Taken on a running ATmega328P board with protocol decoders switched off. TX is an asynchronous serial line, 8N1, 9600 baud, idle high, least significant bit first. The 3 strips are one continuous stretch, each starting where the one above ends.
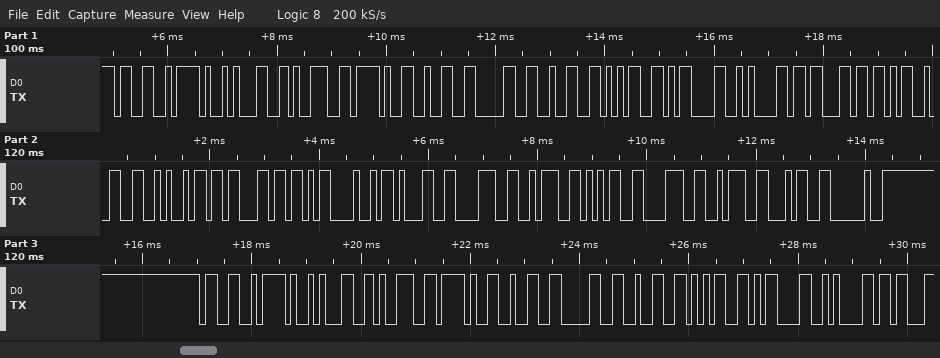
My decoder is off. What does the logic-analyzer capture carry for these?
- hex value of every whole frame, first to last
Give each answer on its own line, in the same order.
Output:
33 2F 31 39 2F 32 30 32 35 0D 0A 1B 5B 32 4A 1B 5B 48 31 38 3A 35 38 3A 34 20 33 2F 31 39 2F 32 30 32 35 0D 0A 1B
